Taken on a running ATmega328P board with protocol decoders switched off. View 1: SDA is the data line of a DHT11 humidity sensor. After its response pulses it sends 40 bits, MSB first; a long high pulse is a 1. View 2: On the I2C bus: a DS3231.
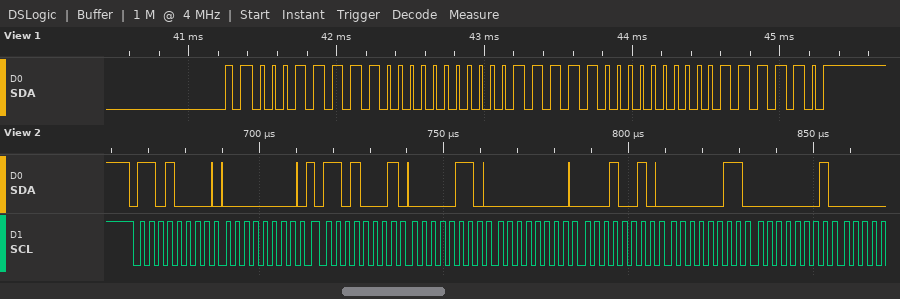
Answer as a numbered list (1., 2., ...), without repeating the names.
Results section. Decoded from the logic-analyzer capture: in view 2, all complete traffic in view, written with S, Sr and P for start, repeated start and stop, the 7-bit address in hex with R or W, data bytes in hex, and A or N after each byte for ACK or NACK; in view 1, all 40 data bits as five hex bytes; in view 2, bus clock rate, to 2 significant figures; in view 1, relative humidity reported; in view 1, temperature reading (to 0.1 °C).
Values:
1. S 68W A 00 A Sr 68R A 06 A 00 A 12 A 03 A 01 A
2. 1F 00 1F 00 3E
3. 400 kHz
4. 31 %
5. 31.0 °C
